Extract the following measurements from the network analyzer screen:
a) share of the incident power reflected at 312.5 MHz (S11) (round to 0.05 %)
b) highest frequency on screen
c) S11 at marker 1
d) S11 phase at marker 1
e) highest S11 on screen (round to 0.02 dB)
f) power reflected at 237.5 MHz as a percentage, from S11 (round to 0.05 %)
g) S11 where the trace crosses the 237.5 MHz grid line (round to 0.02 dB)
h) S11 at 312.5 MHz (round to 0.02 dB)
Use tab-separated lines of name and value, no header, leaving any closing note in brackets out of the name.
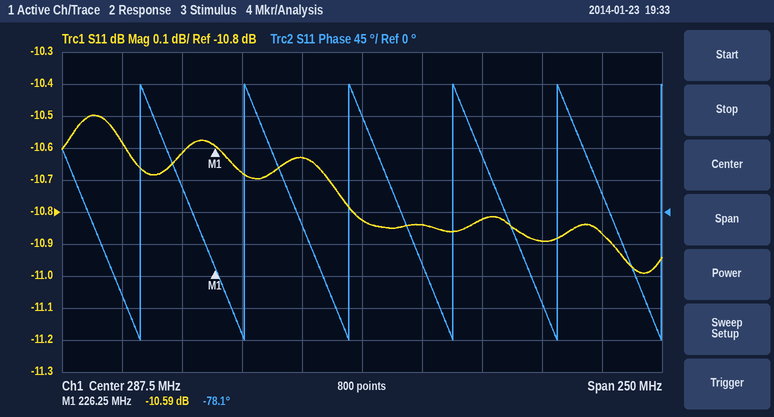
share of the incident power reflected at 312.5 MHz (S11)	8.25 %
highest frequency on screen	412.5 MHz
S11 at marker 1	-10.59 dB
S11 phase at marker 1	-78.1°
highest S11 on screen	-10.50 dB
power reflected at 237.5 MHz as a percentage, from S11	8.55 %
S11 where the trace crosses the 237.5 MHz grid line	-10.68 dB
S11 at 312.5 MHz	-10.84 dB
